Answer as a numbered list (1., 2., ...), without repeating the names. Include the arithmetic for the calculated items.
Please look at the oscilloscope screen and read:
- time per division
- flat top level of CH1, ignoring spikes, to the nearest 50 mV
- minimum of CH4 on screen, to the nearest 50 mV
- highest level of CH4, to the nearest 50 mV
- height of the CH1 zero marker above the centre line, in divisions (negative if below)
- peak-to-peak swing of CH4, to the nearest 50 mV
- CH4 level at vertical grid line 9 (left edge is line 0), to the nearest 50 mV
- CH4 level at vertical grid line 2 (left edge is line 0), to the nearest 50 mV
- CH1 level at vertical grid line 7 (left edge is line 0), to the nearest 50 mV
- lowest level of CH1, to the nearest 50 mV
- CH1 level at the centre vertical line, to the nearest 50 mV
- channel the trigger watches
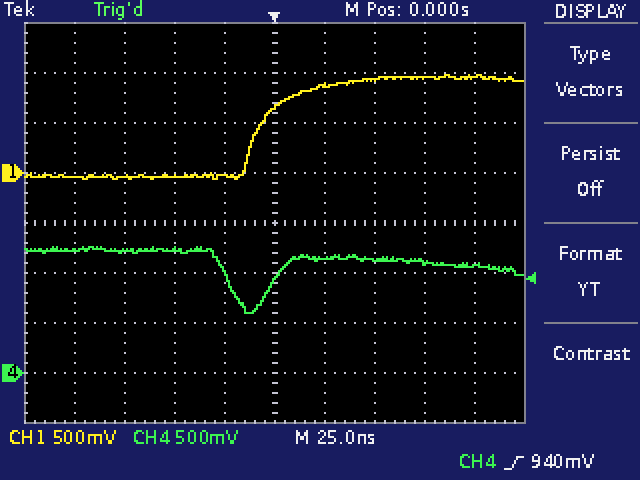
1. 25 ns
2. 950 mV
3. 600 mV
4. 1.25 V
5. +1.0 div
6. 1.25 V − (600 mV) = 650 mV
7. 1.05 V
8. 1.20 V
9. 950 mV
10. -50 mV
11. 650 mV
12. CH4
